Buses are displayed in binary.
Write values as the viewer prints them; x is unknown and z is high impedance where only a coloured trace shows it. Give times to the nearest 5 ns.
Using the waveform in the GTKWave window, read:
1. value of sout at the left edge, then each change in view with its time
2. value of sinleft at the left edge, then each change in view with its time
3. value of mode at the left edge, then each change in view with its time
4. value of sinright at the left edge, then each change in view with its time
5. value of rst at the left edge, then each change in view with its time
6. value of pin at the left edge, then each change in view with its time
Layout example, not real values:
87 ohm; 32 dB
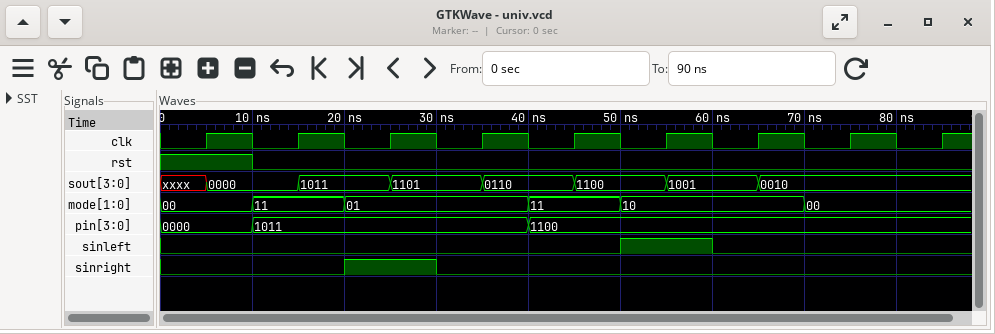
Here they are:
xxxx, 0000 at 5 ns, 1011 at 15 ns, 1101 at 25 ns, 0110 at 35 ns, 1100 at 45 ns, 1001 at 55 ns, 0010 at 65 ns; 0, 1 at 50 ns, 0 at 60 ns; 00, 11 at 10 ns, 01 at 20 ns, 11 at 40 ns, 10 at 50 ns, 00 at 70 ns; 0, 1 at 20 ns, 0 at 30 ns; 1, 0 at 10 ns; 0000, 1011 at 10 ns, 1100 at 40 ns
